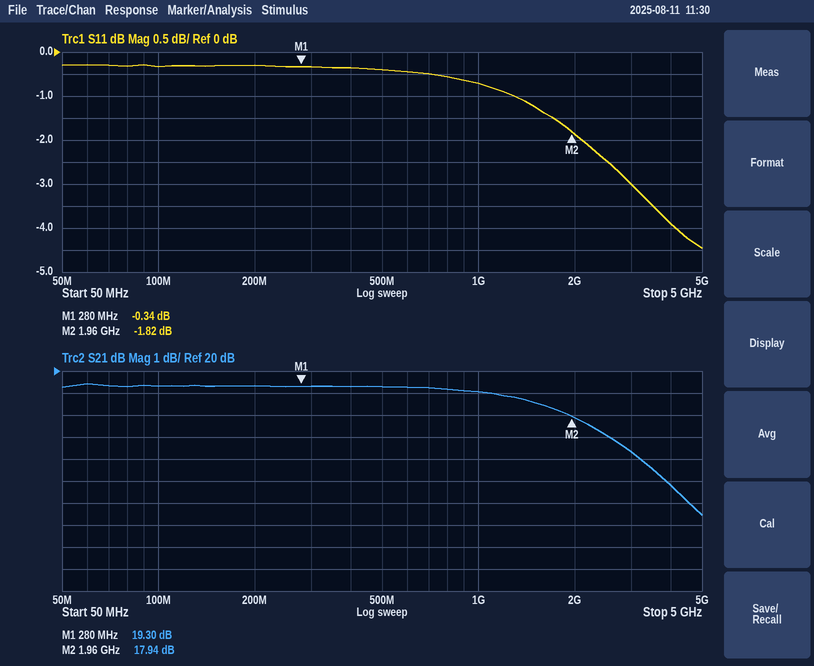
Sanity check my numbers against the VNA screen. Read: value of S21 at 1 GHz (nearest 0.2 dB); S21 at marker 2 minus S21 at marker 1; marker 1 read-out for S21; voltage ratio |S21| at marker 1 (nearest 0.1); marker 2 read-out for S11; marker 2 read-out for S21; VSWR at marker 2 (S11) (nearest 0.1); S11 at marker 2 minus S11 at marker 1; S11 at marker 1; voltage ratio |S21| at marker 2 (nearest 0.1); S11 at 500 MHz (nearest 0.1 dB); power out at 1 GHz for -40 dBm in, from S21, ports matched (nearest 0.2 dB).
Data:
19.0 dB
-1.36 dB
19.30 dB
9.2
-1.82 dB
17.94 dB
9.6
-1.48 dB
-0.34 dB
7.9
-0.4 dB
-21.0 dBm
